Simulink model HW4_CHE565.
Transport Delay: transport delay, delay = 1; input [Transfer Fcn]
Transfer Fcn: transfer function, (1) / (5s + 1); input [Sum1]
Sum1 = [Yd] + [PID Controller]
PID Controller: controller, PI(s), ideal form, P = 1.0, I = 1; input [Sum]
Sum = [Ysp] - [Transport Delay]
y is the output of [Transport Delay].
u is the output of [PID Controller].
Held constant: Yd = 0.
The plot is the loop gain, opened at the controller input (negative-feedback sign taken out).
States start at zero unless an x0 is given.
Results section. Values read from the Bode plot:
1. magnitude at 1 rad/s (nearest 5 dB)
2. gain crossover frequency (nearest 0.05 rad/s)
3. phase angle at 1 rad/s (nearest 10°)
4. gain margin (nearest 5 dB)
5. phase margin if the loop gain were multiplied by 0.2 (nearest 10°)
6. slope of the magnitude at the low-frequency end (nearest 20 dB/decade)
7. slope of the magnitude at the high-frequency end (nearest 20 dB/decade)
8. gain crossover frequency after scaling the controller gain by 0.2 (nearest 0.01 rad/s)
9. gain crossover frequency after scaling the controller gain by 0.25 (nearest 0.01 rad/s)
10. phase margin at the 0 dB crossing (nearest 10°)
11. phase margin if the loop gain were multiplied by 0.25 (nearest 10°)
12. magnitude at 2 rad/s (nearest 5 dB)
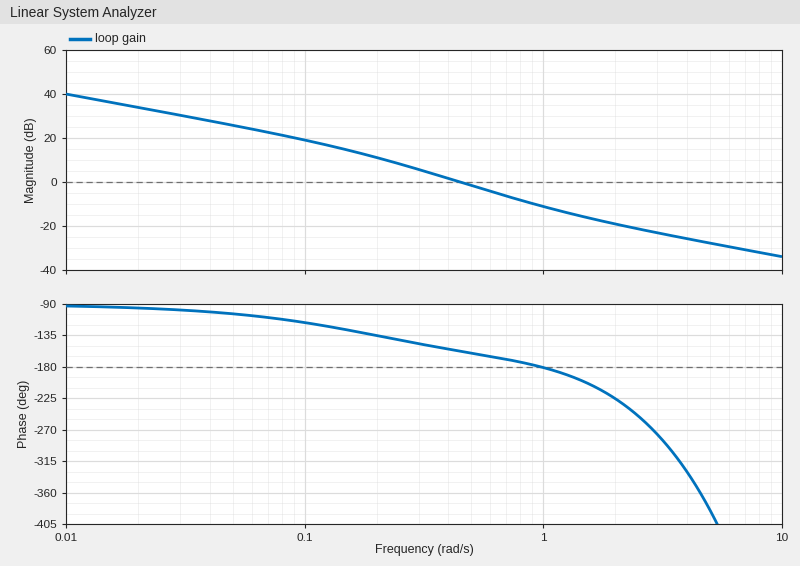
-10 dB
0.45 rad/s
-180°
10 dB
50°
-20 dB/decade
-20 dB/decade
0.16 rad/s
0.19 rad/s
20°
50°
-20 dB
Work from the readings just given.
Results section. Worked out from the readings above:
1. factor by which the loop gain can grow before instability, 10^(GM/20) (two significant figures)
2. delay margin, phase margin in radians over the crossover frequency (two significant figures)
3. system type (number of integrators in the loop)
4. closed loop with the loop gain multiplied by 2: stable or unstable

3.2
0.78 s
1
stable
